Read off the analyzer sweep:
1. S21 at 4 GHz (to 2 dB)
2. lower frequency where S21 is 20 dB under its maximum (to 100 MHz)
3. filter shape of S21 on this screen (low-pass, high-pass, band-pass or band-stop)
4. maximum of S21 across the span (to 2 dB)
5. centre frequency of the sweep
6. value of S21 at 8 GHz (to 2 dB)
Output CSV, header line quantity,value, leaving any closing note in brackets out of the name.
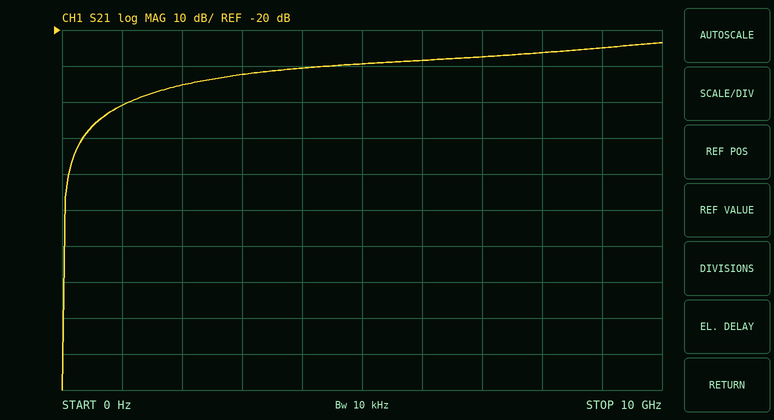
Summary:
quantity,value
S21 at 4 GHz,-30 dB
lower frequency where S21 is 20 dB under its maximum,700 MHz
filter shape of S21 on this screen,high-pass
maximum of S21 across the span,-24 dB
centre frequency of the sweep,5 GHz
value of S21 at 8 GHz,-26 dB
